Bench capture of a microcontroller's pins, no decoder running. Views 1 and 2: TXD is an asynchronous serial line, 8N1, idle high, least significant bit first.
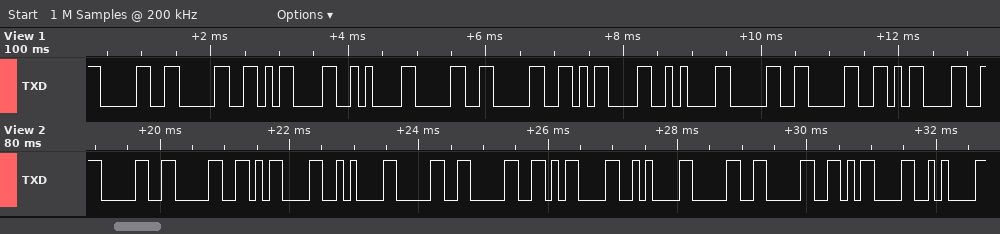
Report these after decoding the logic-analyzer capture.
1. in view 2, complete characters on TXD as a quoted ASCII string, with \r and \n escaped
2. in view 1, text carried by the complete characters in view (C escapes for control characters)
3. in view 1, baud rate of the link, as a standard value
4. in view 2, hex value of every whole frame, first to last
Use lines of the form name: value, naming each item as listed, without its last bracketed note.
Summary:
in view 2, complete characters on TXD as a quoted ASCII string, with \r and \n escaped: "00\r\n00\r\n00\r\n"
in view 1, text carried by the complete characters in view: "00\r\n00\r\n00\r"
in view 1, baud rate of the link, as a standard value: 9600 baud
in view 2, hex value of every whole frame, first to last: 30 30 0D 0A 30 30 0D 0A 30 30 0D 0A
